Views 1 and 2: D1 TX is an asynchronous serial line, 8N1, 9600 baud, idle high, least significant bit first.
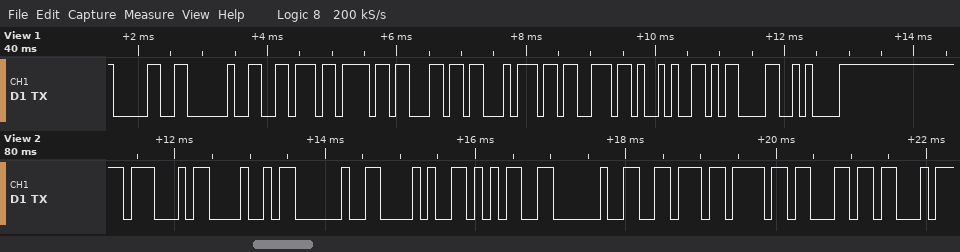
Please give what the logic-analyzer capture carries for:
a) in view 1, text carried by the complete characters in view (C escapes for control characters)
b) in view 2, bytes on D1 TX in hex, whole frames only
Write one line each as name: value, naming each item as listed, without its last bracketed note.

in view 1, text carried by the complete characters in view: "0 volts)\r\n"
in view 2, bytes on D1 TX in hex, whole frames only: 0x47 0x48 0x20 0x28 0x35 0x20 0x76 0x6F 0x6C
